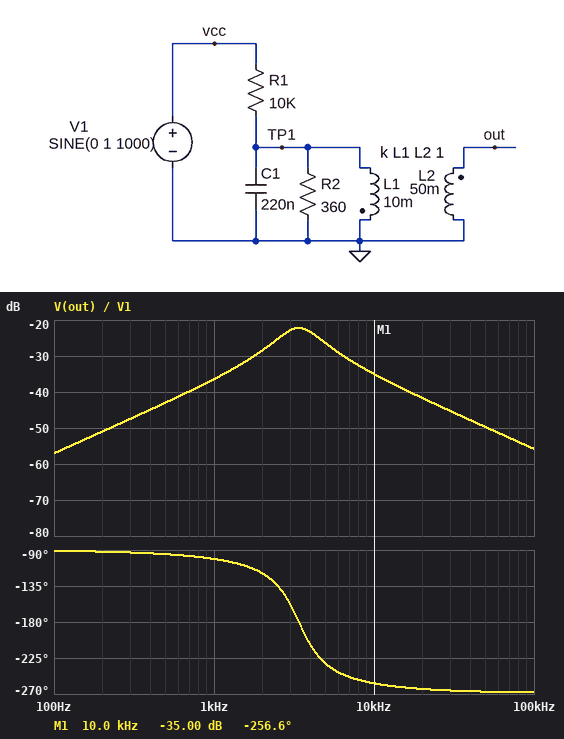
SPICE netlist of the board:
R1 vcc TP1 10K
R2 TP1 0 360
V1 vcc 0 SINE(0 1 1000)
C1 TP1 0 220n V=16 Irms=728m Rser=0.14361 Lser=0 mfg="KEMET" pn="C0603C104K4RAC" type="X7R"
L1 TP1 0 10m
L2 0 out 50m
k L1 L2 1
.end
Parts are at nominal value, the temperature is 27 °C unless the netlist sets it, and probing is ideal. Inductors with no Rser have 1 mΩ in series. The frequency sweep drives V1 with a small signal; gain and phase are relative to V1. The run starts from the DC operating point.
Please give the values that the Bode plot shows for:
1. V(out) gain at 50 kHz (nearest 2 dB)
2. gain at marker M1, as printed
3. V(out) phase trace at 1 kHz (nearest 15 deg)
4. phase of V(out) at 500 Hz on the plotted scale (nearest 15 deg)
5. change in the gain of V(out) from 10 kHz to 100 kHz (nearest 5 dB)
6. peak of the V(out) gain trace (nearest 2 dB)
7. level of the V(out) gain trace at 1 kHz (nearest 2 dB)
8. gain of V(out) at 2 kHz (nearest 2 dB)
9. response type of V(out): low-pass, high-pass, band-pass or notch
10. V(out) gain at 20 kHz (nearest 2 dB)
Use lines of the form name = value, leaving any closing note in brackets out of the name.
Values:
V(out) gain at 50 kHz = -50 dB
gain at marker M1, as printed = -35.00 dB
V(out) phase trace at 1 kHz = -105 deg
phase of V(out) at 500 Hz on the plotted scale = -90 deg
change in the gain of V(out) from 10 kHz to 100 kHz = -20 dB
peak of the V(out) gain trace = -22 dB
level of the V(out) gain trace at 1 kHz = -36 dB
gain of V(out) at 2 kHz = -28 dB
response type of V(out): low-pass, high-pass, band-pass or notch = band-pass
V(out) gain at 20 kHz = -42 dB
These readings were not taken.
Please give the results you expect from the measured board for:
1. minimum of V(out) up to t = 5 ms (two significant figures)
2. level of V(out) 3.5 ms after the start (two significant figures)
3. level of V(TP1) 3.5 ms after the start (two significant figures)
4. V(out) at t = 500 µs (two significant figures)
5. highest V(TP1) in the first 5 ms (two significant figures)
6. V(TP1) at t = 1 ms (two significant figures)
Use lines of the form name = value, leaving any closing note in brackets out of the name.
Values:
minimum of V(out) up to t = 5 ms = -17 mV
level of V(out) 3.5 ms after the start = 15 mV
level of V(TP1) 3.5 ms after the start = -6.6 mV
V(out) at t = 500 µs = 14 mV
highest V(TP1) in the first 5 ms = 7.5 mV
V(TP1) at t = 1 ms = 6.6 mV
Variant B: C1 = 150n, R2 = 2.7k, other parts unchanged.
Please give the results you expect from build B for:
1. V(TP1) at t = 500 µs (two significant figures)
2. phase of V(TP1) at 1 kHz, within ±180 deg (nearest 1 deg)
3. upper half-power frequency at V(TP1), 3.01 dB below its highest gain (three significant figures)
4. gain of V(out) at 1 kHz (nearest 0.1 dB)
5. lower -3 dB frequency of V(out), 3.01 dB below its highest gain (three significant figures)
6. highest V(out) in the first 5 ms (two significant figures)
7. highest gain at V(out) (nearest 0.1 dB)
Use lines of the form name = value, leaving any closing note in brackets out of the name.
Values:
V(TP1) at t = 500 µs = -9.6 mV
phase of V(TP1) at 1 kHz, within ±180 deg = 88 deg
upper half-power frequency at V(TP1), 3.01 dB below its highest gain = 4.37 kHz
gain of V(out) at 1 kHz = -36.5 dB
lower -3 dB frequency of V(out), 3.01 dB below its highest gain = 3.87 kHz
highest V(out) in the first 5 ms = 22 mV
highest gain at V(out) = -6.5 dB
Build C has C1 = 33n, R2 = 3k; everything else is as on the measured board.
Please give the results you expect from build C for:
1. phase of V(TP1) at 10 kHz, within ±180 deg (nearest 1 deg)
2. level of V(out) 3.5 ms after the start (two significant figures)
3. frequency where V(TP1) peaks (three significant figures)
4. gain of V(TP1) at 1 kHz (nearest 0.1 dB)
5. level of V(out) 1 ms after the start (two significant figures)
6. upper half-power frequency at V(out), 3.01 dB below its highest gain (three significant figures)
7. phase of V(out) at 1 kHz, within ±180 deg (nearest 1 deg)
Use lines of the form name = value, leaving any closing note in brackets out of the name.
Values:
phase of V(TP1) at 10 kHz, within ±180 deg = -48 deg
level of V(out) 3.5 ms after the start = 14 mV
frequency where V(TP1) peaks = 8.76 kHz
gain of V(TP1) at 1 kHz = -43.9 dB
level of V(out) 1 ms after the start = -14 mV
upper half-power frequency at V(out), 3.01 dB below its highest gain = 9.87 kHz
phase of V(out) at 1 kHz, within ±180 deg = -92 deg
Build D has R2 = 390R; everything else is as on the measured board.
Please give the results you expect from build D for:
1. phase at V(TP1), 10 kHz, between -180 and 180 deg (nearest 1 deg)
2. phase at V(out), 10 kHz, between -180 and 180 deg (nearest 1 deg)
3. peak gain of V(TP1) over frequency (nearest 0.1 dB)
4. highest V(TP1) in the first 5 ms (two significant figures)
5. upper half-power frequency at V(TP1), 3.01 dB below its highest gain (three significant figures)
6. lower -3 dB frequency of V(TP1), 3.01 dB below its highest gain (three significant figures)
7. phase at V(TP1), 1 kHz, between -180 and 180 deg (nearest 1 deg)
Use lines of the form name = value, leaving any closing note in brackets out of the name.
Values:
phase at V(TP1), 10 kHz, between -180 and 180 deg = -78 deg
phase at V(out), 10 kHz, between -180 and 180 deg = 102 deg
peak gain of V(TP1) over frequency = -28.5 dB
highest V(TP1) in the first 5 ms = 7.7 mV
upper half-power frequency at V(TP1), 3.01 dB below its highest gain = 4.49 kHz
lower -3 dB frequency of V(TP1), 3.01 dB below its highest gain = 2.56 kHz
phase at V(TP1), 1 kHz, between -180 and 180 deg = 80 deg
